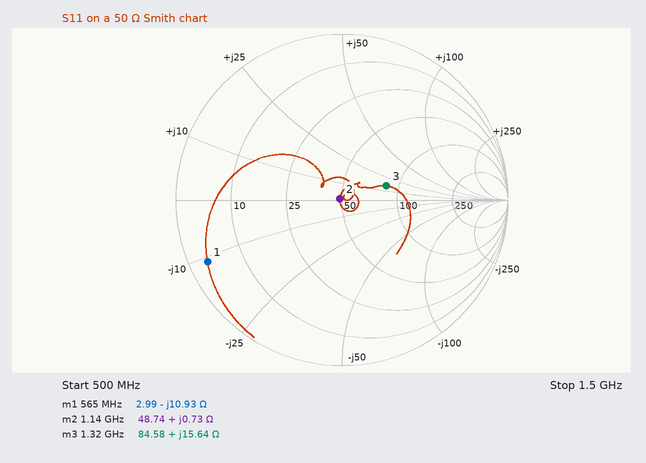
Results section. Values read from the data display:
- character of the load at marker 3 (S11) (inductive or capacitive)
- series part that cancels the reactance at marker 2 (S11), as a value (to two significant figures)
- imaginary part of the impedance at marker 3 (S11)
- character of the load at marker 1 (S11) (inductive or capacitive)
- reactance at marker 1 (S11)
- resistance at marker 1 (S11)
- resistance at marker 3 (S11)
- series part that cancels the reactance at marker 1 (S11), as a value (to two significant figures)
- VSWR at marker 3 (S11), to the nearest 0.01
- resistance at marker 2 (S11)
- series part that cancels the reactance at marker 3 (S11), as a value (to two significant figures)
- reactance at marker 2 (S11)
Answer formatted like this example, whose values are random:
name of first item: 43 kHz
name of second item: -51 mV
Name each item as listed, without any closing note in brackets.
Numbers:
character of the load at marker 3 (S11): inductive
series part that cancels the reactance at marker 2 (S11), as a value: 190 pF
imaginary part of the impedance at marker 3: +15.64 Ω
character of the load at marker 1 (S11): capacitive
reactance at marker 1: -10.93 Ω
resistance at marker 1: 2.99 Ω
resistance at marker 3: 84.58 Ω
series part that cancels the reactance at marker 1 (S11), as a value: 3.1 nH
VSWR at marker 3 (S11), to the nearest 0.01: 1.78
resistance at marker 2: 48.74 Ω
series part that cancels the reactance at marker 3 (S11), as a value: 7.7 pF
reactance at marker 2: +0.73 Ω
